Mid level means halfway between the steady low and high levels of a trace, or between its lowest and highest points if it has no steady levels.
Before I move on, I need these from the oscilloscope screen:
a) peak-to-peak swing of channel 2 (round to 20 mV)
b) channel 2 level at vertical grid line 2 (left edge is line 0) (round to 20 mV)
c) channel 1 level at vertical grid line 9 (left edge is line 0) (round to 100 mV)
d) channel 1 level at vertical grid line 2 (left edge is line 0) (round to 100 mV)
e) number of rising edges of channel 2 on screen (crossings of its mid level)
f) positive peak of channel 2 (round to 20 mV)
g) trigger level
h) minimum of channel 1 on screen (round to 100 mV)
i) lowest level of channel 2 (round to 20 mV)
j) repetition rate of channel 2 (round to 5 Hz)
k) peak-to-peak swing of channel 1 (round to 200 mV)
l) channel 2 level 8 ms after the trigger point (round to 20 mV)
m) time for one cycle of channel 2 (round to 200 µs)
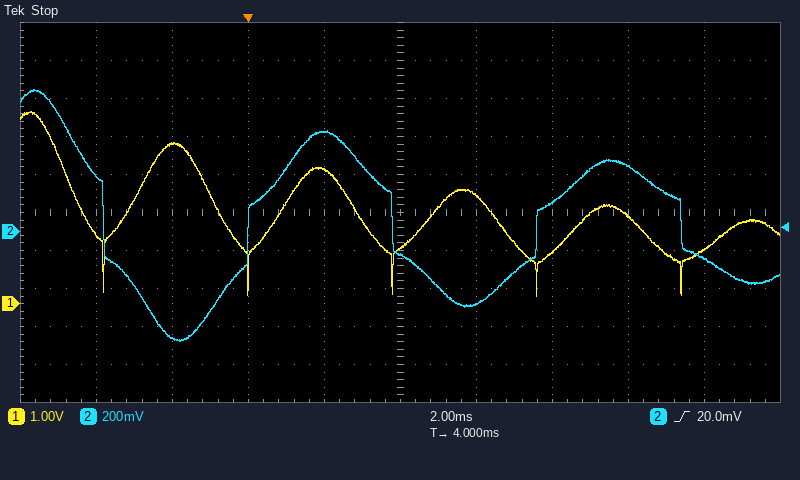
1.32 V
-560 mV
1.4 V
4.2 V
2
740 mV
20.0 mV
200 mV
-580 mV
130 Hz
4.8 V
160 mV
7.6 ms
